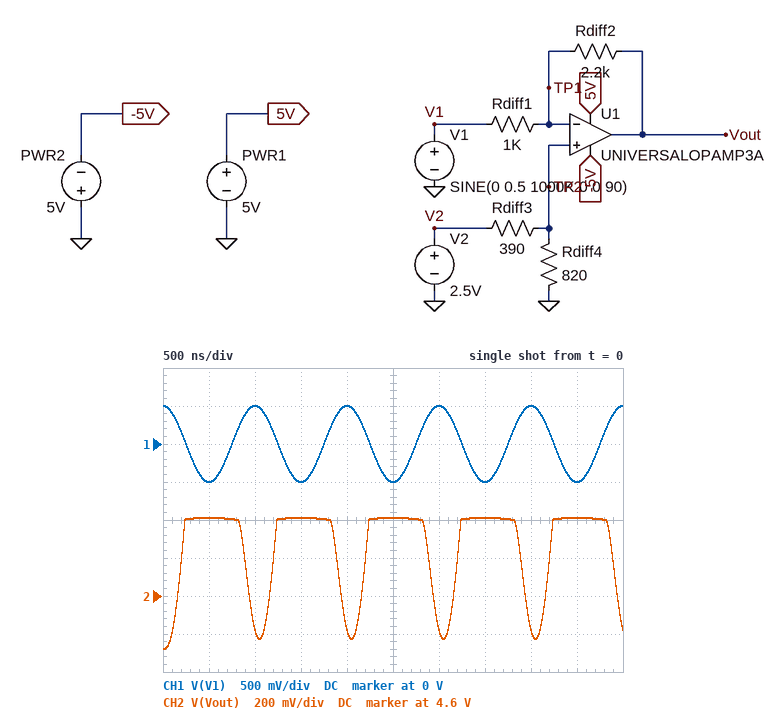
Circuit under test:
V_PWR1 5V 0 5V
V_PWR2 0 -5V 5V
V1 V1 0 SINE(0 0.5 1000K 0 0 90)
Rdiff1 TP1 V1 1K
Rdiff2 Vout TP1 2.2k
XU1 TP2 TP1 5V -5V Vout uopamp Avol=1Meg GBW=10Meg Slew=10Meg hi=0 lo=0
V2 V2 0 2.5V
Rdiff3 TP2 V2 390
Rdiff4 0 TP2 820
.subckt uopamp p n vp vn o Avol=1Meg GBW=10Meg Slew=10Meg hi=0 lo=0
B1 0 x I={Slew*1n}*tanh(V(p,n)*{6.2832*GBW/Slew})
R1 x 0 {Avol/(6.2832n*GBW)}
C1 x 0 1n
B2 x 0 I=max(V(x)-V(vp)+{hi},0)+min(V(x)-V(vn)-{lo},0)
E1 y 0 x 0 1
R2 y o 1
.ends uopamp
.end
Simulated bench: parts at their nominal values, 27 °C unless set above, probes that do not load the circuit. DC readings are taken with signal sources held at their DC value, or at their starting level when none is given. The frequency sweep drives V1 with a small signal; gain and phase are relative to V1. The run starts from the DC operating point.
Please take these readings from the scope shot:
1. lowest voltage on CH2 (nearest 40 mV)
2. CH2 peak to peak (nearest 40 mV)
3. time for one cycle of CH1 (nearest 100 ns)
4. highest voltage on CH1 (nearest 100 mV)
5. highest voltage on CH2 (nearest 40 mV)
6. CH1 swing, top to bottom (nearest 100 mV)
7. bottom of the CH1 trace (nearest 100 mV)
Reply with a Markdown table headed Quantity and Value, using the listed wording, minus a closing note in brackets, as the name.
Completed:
| Quantity | Value |
|---|---|
| lowest voltage on CH2 | 4.32 V |
| CH2 peak to peak | 680 mV |
| time for one cycle of CH1 | 1.0 µs |
| highest voltage on CH1 | 500 mV |
| highest voltage on CH2 | 5.00 V |
| CH1 swing, top to bottom | 1.0 V |
| bottom of the CH1 trace | -500 mV |
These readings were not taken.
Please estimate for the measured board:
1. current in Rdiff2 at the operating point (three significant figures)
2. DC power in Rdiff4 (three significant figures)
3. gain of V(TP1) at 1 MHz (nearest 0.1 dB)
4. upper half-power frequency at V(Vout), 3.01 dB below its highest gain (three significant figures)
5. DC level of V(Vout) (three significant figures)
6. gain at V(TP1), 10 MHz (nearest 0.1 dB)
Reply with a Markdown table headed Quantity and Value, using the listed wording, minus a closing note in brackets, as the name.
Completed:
| Quantity | Value |
|---|---|
| current in Rdiff2 at the operating point | 1.19 mA |
| DC power in Rdiff4 | 3.50 mW |
| gain of V(TP1) at 1 MHz | -13.6 dB |
| upper half-power frequency at V(Vout), 3.01 dB below its highest gain | 3.12 MHz |
| DC level of V(Vout) | 4.32 V |
| gain at V(TP1), 10 MHz | -3.7 dB |
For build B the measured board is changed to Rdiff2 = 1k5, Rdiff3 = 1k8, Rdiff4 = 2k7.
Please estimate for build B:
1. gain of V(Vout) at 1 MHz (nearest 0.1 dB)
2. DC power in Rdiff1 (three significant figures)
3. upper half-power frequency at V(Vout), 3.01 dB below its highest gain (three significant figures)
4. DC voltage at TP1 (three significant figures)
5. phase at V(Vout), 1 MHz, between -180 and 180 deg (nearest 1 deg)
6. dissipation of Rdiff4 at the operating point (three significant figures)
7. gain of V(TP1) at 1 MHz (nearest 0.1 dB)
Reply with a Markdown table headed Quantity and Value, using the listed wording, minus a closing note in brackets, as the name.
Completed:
| Quantity | Value |
|---|---|
| gain of V(Vout) at 1 MHz | 3.3 dB |
| DC power in Rdiff1 | 1.00 mW |
| upper half-power frequency at V(Vout), 3.01 dB below its highest gain | 4.00 MHz |
| DC voltage at TP1 | 1.50 V |
| phase at V(Vout), 1 MHz, between -180 and 180 deg | 166 deg |
| dissipation of Rdiff4 at the operating point | 833 µW |
| gain of V(TP1) at 1 MHz | -16.7 dB |
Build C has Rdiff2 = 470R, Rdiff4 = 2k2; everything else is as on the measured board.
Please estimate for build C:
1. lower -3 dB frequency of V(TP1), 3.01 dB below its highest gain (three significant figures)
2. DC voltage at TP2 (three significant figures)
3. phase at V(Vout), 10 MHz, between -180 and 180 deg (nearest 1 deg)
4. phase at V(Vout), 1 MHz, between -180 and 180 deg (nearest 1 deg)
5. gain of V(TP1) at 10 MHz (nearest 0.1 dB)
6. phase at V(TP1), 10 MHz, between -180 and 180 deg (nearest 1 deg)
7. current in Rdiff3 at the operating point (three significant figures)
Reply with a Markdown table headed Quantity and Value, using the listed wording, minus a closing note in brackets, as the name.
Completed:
| Quantity | Value |
|---|---|
| lower -3 dB frequency of V(TP1), 3.01 dB below its highest gain | 6.80 MHz |
| DC voltage at TP2 | 2.12 V |
| phase at V(Vout), 10 MHz, between -180 and 180 deg | 124 deg |
| phase at V(Vout), 1 MHz, between -180 and 180 deg | 172 deg |
| gain of V(TP1) at 10 MHz | -11.5 dB |
| phase at V(TP1), 10 MHz, between -180 and 180 deg | 34 deg |
| current in Rdiff3 at the operating point | 965 µA |
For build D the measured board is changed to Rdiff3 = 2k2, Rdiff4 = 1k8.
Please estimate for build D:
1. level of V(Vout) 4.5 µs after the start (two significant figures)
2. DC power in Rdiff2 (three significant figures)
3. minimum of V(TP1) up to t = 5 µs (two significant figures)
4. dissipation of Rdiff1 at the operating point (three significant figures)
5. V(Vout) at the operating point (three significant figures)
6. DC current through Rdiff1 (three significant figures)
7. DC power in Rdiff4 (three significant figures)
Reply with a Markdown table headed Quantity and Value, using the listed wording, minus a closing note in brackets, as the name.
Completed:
| Quantity | Value |
|---|---|
| level of V(Vout) 4.5 µs after the start | 4.6 V |
| DC power in Rdiff2 | 859 µW |
| minimum of V(TP1) up to t = 5 µs | 1.0 V |
| dissipation of Rdiff1 at the operating point | 391 µW |
| V(Vout) at the operating point | 2.50 V |
| DC current through Rdiff1 | 625 µA |
| DC power in Rdiff4 | 703 µW |
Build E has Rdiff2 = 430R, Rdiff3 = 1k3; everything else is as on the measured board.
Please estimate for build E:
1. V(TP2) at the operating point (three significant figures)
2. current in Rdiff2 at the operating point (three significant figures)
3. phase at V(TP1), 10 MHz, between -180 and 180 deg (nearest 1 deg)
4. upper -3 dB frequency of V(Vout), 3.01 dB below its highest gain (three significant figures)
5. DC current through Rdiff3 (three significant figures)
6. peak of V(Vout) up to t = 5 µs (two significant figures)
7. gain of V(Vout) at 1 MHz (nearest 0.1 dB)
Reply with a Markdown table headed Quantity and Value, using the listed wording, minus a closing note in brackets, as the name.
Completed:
| Quantity | Value |
|---|---|
| V(TP2) at the operating point | 967 mV |
| current in Rdiff2 at the operating point | 467 µA |
| phase at V(TP1), 10 MHz, between -180 and 180 deg | 35 deg |
| upper -3 dB frequency of V(Vout), 3.01 dB below its highest gain | 6.99 MHz |
| DC current through Rdiff3 | 1.18 mA |
| peak of V(Vout) up to t = 5 µs | 1.6 V |
| gain of V(Vout) at 1 MHz | -7.4 dB |
